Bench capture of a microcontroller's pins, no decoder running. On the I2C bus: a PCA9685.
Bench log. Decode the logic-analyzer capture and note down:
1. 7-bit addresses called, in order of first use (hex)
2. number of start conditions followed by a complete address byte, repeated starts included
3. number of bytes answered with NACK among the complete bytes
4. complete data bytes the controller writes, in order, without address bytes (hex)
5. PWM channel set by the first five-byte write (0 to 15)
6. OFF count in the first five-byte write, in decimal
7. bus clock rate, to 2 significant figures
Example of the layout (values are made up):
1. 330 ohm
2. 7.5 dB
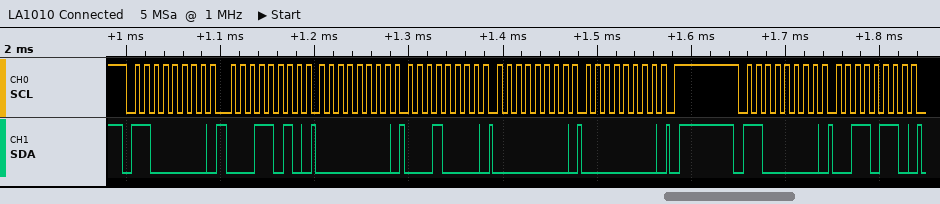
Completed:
1. 0x60
2. 2
3. 0
4. 1A 00 10 00 00 36
5. 5
6. 0
7. 100 kHz
